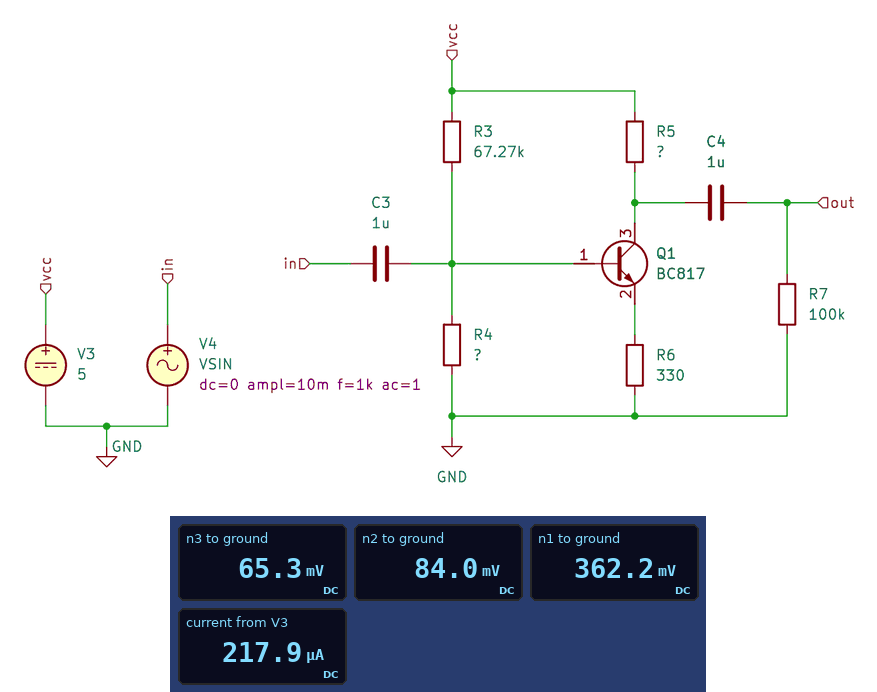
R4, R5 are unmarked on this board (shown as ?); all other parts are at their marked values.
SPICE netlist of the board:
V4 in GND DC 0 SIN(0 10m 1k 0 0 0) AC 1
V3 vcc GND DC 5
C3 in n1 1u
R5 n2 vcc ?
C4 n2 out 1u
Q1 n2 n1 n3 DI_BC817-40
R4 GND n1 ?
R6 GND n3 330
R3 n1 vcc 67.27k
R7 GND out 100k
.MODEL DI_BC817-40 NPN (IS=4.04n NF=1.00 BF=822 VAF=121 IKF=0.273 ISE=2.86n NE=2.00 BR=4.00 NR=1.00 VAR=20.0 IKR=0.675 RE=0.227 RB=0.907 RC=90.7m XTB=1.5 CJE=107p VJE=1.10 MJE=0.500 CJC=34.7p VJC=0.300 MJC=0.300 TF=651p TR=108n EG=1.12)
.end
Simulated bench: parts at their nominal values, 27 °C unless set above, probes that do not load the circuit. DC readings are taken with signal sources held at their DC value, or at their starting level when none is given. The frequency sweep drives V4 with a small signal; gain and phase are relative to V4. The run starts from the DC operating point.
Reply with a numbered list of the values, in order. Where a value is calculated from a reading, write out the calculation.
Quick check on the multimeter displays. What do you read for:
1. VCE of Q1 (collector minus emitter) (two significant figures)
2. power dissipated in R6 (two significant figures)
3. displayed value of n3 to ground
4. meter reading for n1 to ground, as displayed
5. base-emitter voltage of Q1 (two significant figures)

1. 84 mV - 65.3 mV = 19 mV
2. (65.3 mV)^2 / 330 Ω = 13 µW
3. 65.3 mV
4. 362.2 mV
5. 362.2 mV - 65.3 mV = 300 mV
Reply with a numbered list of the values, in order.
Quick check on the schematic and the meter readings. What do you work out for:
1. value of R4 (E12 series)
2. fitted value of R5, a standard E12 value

1. 18 kΩ
2. 33 kΩ
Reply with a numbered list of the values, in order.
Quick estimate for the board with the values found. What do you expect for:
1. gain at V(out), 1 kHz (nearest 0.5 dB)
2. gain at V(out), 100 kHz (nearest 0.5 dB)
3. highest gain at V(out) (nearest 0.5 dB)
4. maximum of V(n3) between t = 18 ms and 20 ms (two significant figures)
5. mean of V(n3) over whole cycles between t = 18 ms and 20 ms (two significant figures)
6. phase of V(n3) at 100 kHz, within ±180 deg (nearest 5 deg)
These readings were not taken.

1. -15.0 dB
2. -12.0 dB
3. 0 dB
4. 70 mV
5. 65 mV
6. 5 deg
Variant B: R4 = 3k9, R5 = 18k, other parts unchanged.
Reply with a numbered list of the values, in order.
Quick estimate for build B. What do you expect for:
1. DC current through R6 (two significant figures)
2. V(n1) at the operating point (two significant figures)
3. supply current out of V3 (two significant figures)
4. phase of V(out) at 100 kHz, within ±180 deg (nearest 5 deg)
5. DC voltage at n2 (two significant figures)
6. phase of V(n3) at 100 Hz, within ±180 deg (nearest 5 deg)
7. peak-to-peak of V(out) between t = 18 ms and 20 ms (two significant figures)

1. 66 µA
2. 270 mV
3. 140 µA
4. 170 deg
5. 3.8 V
6. 25 deg
7. 420 mV
